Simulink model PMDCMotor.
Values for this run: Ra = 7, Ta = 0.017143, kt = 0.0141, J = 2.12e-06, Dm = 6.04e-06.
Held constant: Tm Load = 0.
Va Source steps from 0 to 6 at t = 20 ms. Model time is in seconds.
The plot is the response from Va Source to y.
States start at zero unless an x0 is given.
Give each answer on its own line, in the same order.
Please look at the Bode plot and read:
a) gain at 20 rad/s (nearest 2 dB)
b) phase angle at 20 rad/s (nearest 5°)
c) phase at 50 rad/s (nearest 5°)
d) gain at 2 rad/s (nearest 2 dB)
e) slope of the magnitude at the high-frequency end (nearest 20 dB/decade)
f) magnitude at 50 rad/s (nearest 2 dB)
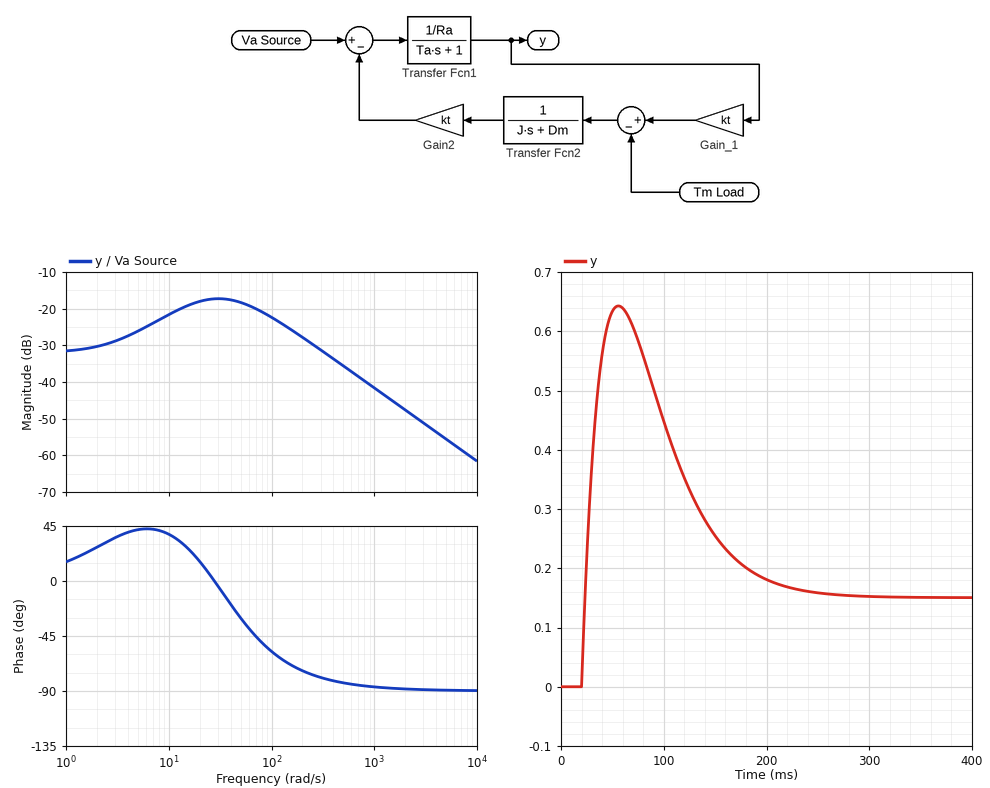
-18 dB
15°
-30°
-30 dB
-20 dB/decade
-18 dB
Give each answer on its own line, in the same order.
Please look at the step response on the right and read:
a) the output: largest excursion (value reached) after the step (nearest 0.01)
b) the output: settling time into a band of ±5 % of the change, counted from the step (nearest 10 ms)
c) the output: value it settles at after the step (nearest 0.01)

0.64
230 ms
0.15
